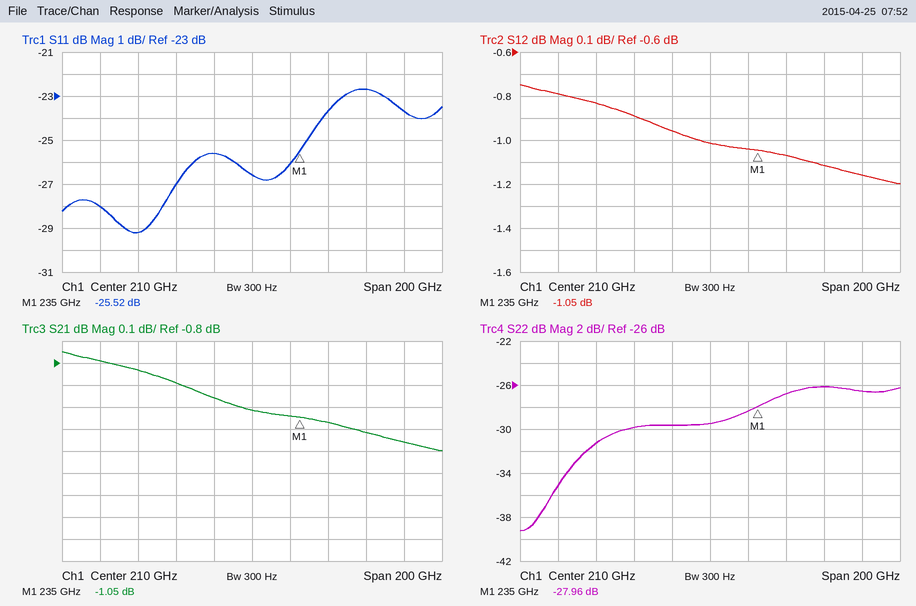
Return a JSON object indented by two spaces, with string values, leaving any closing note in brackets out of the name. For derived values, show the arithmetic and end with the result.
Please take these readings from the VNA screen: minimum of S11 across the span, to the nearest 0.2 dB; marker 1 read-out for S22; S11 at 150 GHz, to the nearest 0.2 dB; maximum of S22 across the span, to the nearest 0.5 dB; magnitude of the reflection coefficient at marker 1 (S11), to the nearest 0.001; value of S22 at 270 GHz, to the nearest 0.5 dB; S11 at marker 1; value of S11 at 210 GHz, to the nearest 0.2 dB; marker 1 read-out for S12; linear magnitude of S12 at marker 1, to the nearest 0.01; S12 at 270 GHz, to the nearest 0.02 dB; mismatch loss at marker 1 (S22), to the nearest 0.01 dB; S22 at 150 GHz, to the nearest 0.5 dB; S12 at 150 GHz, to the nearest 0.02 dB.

{
  "minimum of S11 across the span, to the nearest 0.2 dB": "-29.2 dB",
  "marker 1 read-out for S22": "-27.96 dB",
  "S11 at 150 GHz, to the nearest 0.2 dB": "-29.2 dB",
  "maximum of S22 across the span, to the nearest 0.5 dB": "-26.0 dB",
  "magnitude of the reflection coefficient at marker 1 (S11), to the nearest 0.001": "10^(-25.52/20) ≈ 0.053",
  "value of S22 at 270 GHz, to the nearest 0.5 dB": "-26.0 dB",
  "S11 at marker 1": "-25.52 dB",
  "value of S11 at 210 GHz, to the nearest 0.2 dB": "-26.6 dB",
  "marker 1 read-out for S12": "-1.05 dB",
  "linear magnitude of S12 at marker 1, to the nearest 0.01": "10^(-1.05/20) ≈ 0.89",
  "S12 at 270 GHz, to the nearest 0.02 dB": "-1.12 dB",
  "mismatch loss at marker 1 (S22), to the nearest 0.01 dB": "−10 log10(1 − 10^(-27.96/10)) ≈ 0.01 dB",
  "S22 at 150 GHz, to the nearest 0.5 dB": "-31.5 dB",
  "S12 at 150 GHz, to the nearest 0.02 dB": "-0.84 dB"
}
